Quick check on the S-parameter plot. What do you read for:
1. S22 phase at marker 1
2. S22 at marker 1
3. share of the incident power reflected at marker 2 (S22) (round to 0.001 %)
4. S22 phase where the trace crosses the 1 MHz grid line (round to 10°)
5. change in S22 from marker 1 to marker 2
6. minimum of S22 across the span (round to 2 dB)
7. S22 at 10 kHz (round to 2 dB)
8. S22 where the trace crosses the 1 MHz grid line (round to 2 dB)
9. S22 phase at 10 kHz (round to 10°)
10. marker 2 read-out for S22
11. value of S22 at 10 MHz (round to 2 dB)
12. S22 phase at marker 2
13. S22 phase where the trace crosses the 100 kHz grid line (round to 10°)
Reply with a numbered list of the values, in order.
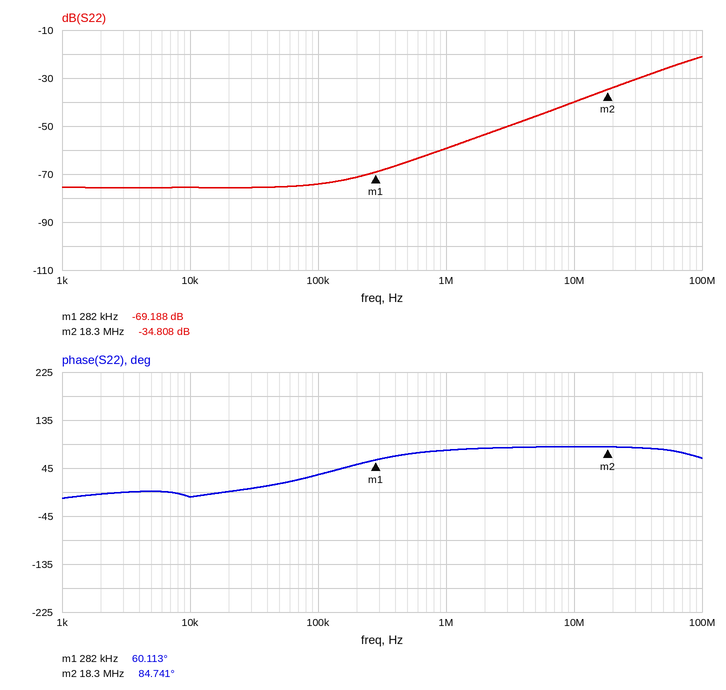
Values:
1. 60.113°
2. -69.188 dB
3. 0.033 %
4. 80°
5. 34.380 dB
6. -76 dB
7. -76 dB
8. -60 dB
9. -10°
10. -34.808 dB
11. -40 dB
12. 84.741°
13. 30°
